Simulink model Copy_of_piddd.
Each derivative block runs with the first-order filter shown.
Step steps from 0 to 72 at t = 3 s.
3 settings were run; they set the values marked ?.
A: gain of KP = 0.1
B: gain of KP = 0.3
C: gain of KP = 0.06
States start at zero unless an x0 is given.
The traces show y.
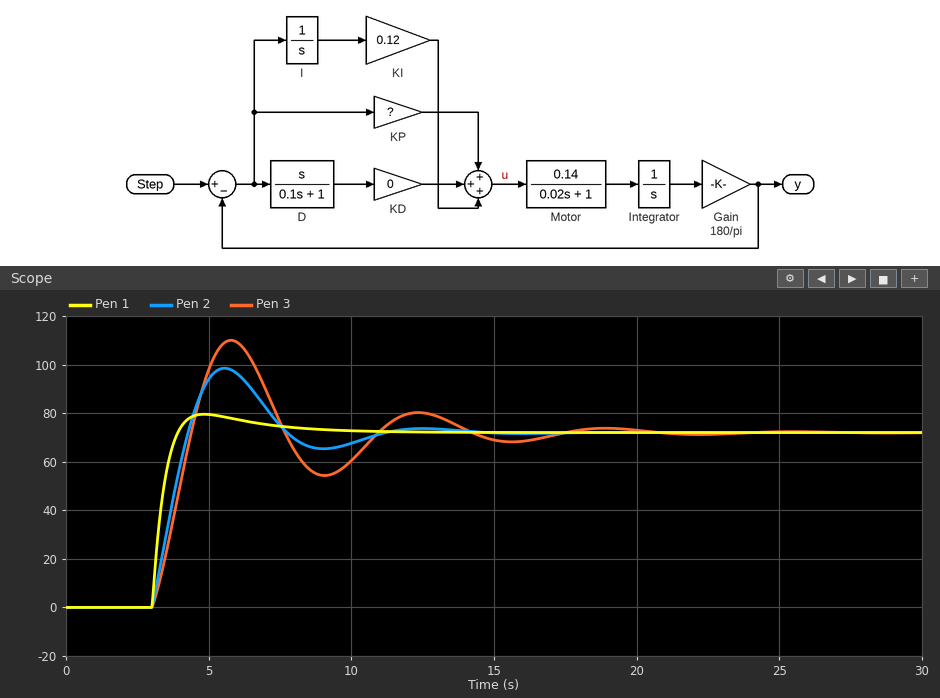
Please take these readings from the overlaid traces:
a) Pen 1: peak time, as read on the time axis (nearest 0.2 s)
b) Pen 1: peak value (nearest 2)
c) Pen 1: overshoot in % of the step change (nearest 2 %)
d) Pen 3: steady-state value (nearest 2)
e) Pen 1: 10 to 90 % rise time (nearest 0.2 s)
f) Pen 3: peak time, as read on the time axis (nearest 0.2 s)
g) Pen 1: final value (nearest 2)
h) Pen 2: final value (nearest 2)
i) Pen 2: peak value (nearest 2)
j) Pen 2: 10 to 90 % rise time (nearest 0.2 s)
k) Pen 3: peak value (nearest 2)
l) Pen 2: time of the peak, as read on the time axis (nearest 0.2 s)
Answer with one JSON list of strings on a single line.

["4.8 s", "80", "10 %", "72", "0.6 s", "5.8 s", "72", "72", "98", "1.0 s", "110", "5.6 s"]
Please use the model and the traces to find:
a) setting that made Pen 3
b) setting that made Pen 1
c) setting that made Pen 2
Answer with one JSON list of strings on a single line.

["C", "B", "A"]
